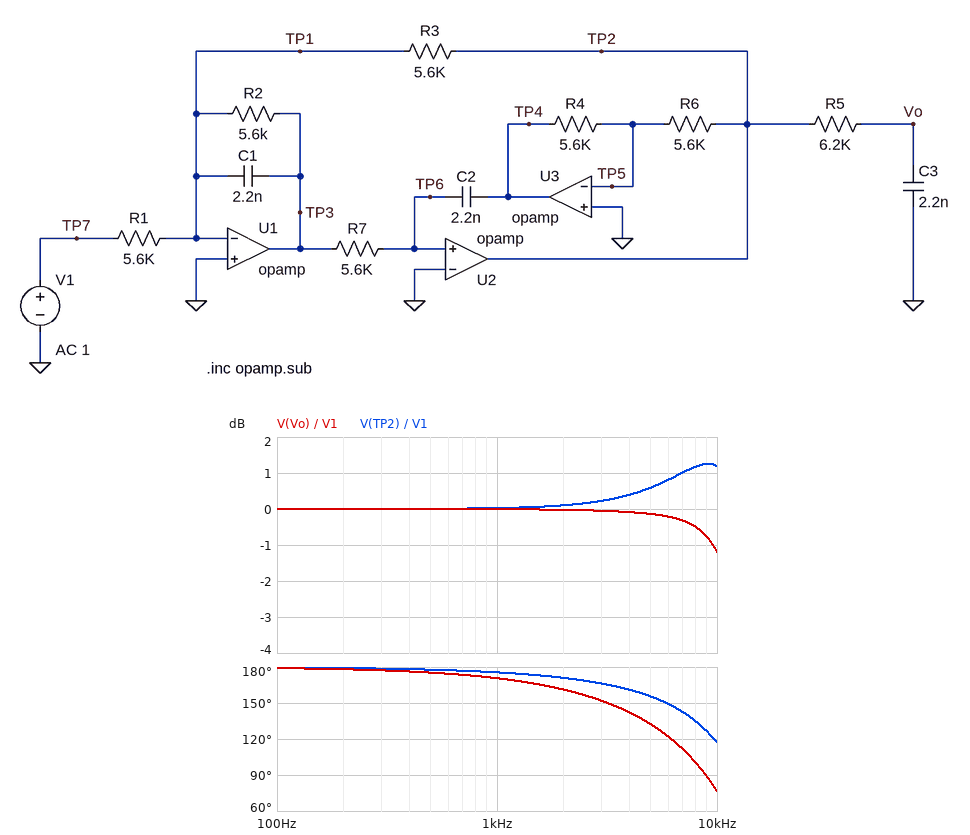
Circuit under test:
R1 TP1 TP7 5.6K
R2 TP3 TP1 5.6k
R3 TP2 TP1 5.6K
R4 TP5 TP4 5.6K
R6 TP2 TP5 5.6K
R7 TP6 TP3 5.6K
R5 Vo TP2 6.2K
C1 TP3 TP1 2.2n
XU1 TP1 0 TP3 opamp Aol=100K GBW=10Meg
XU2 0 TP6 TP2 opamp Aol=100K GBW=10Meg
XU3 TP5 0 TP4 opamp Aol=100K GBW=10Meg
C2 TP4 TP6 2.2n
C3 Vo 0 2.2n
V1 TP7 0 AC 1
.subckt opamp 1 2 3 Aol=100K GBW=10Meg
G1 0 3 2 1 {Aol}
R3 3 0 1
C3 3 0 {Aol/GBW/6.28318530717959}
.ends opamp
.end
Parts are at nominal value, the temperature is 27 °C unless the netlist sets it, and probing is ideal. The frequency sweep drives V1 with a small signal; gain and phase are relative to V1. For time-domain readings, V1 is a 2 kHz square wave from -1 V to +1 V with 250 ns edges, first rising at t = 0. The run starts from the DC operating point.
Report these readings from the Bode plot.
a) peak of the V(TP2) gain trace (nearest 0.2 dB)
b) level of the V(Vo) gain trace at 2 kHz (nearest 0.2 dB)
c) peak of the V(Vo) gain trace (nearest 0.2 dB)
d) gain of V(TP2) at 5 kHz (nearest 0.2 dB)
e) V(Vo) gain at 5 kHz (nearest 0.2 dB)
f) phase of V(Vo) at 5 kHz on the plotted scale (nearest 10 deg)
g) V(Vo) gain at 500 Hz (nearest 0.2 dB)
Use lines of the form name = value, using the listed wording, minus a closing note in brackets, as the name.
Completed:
peak of the V(TP2) gain trace = 1.2 dB
level of the V(Vo) gain trace at 2 kHz = 0 dB
peak of the V(Vo) gain trace = 0 dB
gain of V(TP2) at 5 kHz = 0.6 dB
V(Vo) gain at 5 kHz = -0.2 dB
phase of V(Vo) at 5 kHz on the plotted scale = 130 deg
V(Vo) gain at 500 Hz = 0 dB
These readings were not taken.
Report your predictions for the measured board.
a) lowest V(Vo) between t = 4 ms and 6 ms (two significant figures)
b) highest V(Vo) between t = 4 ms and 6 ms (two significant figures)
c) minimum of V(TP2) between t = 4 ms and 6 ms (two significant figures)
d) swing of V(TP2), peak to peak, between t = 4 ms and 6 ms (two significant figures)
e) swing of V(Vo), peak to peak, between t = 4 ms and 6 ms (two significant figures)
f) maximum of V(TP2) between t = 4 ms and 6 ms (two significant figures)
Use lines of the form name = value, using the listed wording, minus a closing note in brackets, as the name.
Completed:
lowest V(Vo) between t = 4 ms and 6 ms = -1.1 V
highest V(Vo) between t = 4 ms and 6 ms = 1.1 V
minimum of V(TP2) between t = 4 ms and 6 ms = -1.3 V
swing of V(TP2), peak to peak, between t = 4 ms and 6 ms = 2.7 V
swing of V(Vo), peak to peak, between t = 4 ms and 6 ms = 2.3 V
maximum of V(TP2) between t = 4 ms and 6 ms = 1.3 V
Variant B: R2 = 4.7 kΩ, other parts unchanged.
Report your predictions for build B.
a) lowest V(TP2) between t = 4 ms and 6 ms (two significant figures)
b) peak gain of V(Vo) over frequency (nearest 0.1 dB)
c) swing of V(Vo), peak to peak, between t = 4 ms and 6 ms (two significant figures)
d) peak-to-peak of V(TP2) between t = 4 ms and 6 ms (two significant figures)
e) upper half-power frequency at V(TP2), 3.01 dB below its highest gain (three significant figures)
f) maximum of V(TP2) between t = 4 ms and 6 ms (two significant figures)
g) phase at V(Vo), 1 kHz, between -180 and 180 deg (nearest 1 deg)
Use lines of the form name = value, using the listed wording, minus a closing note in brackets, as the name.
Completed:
lowest V(TP2) between t = 4 ms and 6 ms = -1.2 V
peak gain of V(Vo) over frequency = 0 dB
swing of V(Vo), peak to peak, between t = 4 ms and 6 ms = 2.1 V
peak-to-peak of V(TP2) between t = 4 ms and 6 ms = 2.4 V
upper half-power frequency at V(TP2), 3.01 dB below its highest gain = 14.4 kHz
maximum of V(TP2) between t = 4 ms and 6 ms = 1.2 V
phase at V(Vo), 1 kHz, between -180 and 180 deg = 170 deg
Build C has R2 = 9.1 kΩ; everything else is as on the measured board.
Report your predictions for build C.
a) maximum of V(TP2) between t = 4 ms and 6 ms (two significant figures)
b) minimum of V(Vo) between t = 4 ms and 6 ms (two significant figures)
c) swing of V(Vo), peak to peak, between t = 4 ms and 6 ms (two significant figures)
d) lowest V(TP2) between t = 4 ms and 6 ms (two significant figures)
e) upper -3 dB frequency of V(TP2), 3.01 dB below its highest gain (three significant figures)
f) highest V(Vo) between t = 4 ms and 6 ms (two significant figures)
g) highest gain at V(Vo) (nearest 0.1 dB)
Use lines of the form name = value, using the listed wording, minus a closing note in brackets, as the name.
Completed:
maximum of V(TP2) between t = 4 ms and 6 ms = 1.7 V
minimum of V(Vo) between t = 4 ms and 6 ms = -1.4 V
swing of V(Vo), peak to peak, between t = 4 ms and 6 ms = 2.8 V
lowest V(TP2) between t = 4 ms and 6 ms = -1.7 V
upper -3 dB frequency of V(TP2), 3.01 dB below its highest gain = 15.2 kHz
highest V(Vo) between t = 4 ms and 6 ms = 1.4 V
highest gain at V(Vo) = 1.8 dB
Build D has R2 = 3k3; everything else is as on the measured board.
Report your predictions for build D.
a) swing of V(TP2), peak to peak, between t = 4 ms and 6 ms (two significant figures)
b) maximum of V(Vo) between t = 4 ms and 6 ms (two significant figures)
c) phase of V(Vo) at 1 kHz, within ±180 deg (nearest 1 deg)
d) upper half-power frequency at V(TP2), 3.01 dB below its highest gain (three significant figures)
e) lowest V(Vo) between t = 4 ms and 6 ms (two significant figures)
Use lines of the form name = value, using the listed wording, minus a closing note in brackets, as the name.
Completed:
swing of V(TP2), peak to peak, between t = 4 ms and 6 ms = 2.0 V
maximum of V(Vo) between t = 4 ms and 6 ms = 1.0 V
phase of V(Vo) at 1 kHz, within ±180 deg = 168 deg
upper half-power frequency at V(TP2), 3.01 dB below its highest gain = 10.4 kHz
lowest V(Vo) between t = 4 ms and 6 ms = -1.0 V
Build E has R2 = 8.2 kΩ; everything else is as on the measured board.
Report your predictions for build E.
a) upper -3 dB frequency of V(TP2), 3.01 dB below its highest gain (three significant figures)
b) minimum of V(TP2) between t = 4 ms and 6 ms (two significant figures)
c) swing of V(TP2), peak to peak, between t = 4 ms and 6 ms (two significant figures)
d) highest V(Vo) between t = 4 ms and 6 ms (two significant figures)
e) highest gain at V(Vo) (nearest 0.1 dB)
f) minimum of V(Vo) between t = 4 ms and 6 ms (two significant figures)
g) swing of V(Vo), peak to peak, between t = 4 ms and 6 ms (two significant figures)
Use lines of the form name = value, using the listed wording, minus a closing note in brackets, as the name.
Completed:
upper -3 dB frequency of V(TP2), 3.01 dB below its highest gain = 15.3 kHz
minimum of V(TP2) between t = 4 ms and 6 ms = -1.6 V
swing of V(TP2), peak to peak, between t = 4 ms and 6 ms = 3.3 V
highest V(Vo) between t = 4 ms and 6 ms = 1.3 V
highest gain at V(Vo) = 1.2 dB
minimum of V(Vo) between t = 4 ms and 6 ms = -1.3 V
swing of V(Vo), peak to peak, between t = 4 ms and 6 ms = 2.7 V
